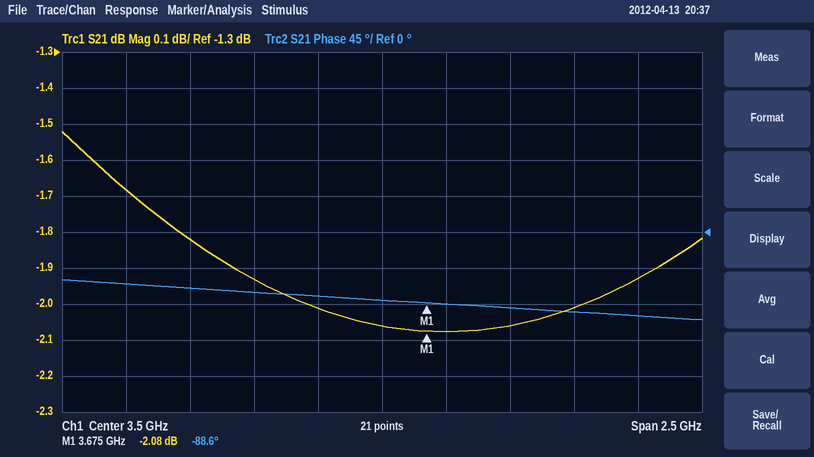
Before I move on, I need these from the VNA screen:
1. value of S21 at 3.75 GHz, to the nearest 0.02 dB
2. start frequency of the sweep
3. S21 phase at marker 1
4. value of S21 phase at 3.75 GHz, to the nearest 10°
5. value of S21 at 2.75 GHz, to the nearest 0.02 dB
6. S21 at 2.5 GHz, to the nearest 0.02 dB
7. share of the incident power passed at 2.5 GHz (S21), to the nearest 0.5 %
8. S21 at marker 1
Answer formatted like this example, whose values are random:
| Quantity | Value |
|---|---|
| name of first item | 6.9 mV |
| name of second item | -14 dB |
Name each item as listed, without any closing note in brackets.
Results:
| Quantity | Value |
|---|---|
| value of S21 at 3.75 GHz, to the nearest 0.02 dB | -2.08 dB |
| start frequency of the sweep | 2.25 GHz |
| S21 phase at marker 1 | -88.6° |
| value of S21 phase at 3.75 GHz, to the nearest 10° | -90° |
| value of S21 at 2.75 GHz, to the nearest 0.02 dB | -1.82 dB |
| S21 at 2.5 GHz, to the nearest 0.02 dB | -1.68 dB |
| share of the incident power passed at 2.5 GHz (S21), to the nearest 0.5 % | 68.0 % |
| S21 at marker 1 | -2.08 dB |
